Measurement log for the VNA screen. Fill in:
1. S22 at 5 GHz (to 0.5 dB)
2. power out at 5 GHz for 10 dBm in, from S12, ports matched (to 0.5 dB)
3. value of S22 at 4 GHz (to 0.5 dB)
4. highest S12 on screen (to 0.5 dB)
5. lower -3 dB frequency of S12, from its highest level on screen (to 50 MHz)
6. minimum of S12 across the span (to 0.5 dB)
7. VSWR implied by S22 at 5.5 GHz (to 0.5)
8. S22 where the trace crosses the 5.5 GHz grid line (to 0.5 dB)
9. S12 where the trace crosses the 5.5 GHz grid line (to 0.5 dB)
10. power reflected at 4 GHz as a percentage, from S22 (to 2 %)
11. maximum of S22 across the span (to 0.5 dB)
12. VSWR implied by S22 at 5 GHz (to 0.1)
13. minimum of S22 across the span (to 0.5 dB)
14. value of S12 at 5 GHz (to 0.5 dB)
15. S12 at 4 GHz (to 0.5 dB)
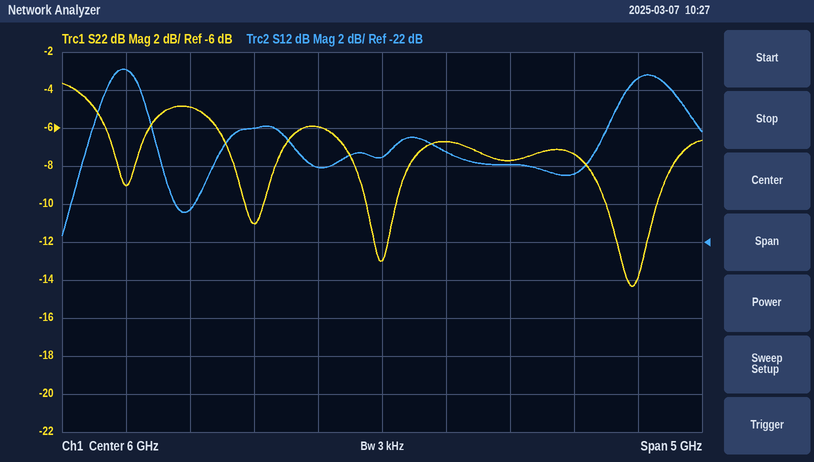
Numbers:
-11.0 dB
-6.0 dBm
-9.0 dB
-13.0 dB
3.75 GHz
-21.5 dB
3.0
-6.0 dB
-18.0 dB
12 %
-3.5 dB
1.8
-14.5 dB
-16.0 dB
-13.0 dB
